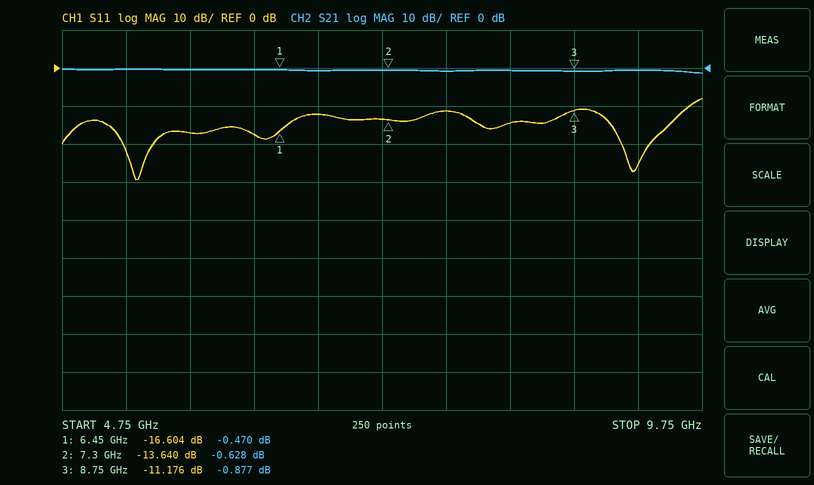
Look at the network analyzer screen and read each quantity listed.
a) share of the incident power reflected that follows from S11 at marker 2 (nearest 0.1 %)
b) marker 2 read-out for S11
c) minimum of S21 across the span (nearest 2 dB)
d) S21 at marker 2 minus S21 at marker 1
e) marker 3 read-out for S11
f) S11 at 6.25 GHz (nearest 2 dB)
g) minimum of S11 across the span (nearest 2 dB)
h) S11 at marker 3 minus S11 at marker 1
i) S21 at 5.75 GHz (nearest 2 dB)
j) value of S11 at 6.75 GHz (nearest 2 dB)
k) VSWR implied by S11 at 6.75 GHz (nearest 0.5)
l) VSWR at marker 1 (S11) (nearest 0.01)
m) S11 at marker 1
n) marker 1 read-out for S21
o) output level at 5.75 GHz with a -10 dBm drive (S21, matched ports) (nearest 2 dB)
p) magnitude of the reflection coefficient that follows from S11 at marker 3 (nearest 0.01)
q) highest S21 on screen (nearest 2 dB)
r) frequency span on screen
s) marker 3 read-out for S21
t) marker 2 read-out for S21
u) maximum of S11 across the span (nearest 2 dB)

4.3 %
-13.640 dB
-2 dB
-0.158 dB
-11.176 dB
-18 dB
-30 dB
5.428 dB
0 dB
-12 dB
1.5
1.35
-16.604 dB
-0.470 dB
-10 dBm
0.28
0 dB
5 GHz
-0.877 dB
-0.628 dB
-8 dB
